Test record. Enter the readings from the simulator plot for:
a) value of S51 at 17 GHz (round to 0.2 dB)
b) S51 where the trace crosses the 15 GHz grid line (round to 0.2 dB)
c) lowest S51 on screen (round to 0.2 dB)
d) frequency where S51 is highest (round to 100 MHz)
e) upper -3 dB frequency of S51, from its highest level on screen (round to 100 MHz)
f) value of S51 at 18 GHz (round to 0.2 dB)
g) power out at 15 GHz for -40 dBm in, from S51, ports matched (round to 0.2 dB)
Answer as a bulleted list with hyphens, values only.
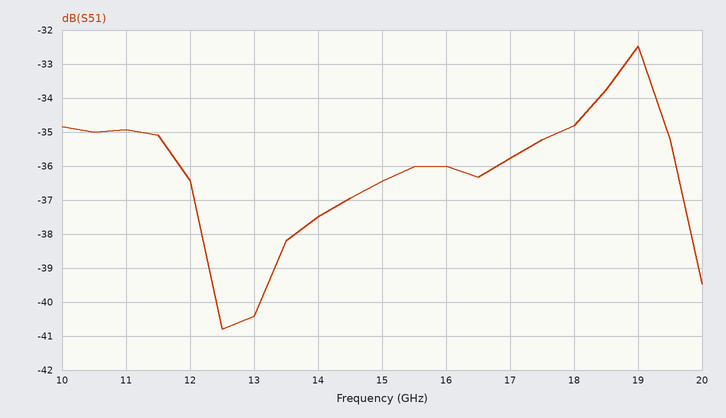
- -35.8 dB
- -36.4 dB
- -40.8 dB
- 19.0 GHz
- 19.5 GHz
- -34.8 dB
- -76.4 dBm
